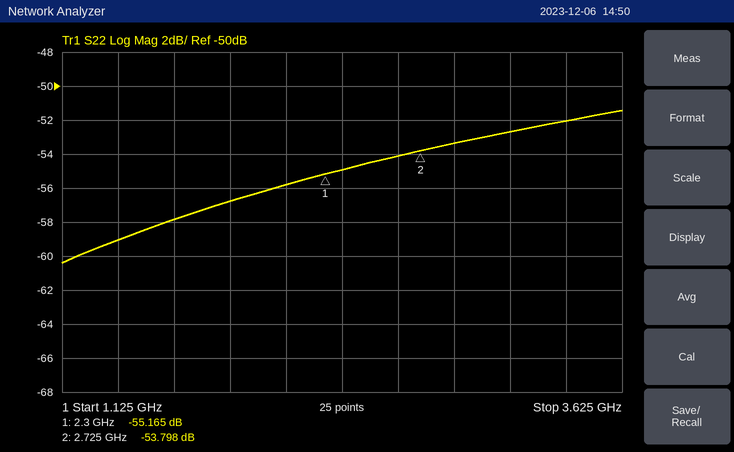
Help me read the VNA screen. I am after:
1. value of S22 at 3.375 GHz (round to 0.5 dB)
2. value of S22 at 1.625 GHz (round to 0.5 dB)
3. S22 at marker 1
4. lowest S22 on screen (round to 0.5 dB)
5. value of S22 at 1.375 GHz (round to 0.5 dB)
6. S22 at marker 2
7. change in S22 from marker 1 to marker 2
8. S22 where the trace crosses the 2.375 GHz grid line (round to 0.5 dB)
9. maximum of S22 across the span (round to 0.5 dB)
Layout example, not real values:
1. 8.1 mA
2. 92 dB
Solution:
1. -52.0 dB
2. -58.0 dB
3. -55.165 dB
4. -60.5 dB
5. -59.0 dB
6. -53.798 dB
7. 1.367 dB
8. -55.0 dB
9. -51.5 dB
